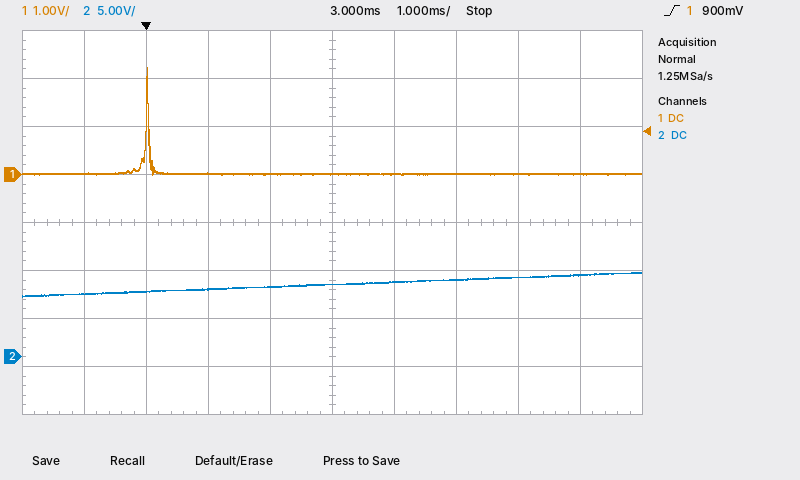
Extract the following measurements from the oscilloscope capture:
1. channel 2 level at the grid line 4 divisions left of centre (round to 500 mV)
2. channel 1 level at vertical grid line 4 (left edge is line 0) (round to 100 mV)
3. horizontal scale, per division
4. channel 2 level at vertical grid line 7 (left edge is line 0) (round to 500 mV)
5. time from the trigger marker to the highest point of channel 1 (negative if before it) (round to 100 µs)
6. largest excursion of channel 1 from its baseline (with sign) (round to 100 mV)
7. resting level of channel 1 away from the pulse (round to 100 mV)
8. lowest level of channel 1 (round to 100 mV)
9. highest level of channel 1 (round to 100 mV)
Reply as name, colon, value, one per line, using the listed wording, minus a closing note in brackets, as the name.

channel 2 level at the grid line 4 divisions left of centre: 6.5 V
channel 1 level at vertical grid line 4 (left edge is line 0): 0.0 V
horizontal scale, per division: 1 ms
channel 2 level at vertical grid line 7 (left edge is line 0): 8.0 V
time from the trigger marker to the highest point of channel 1 (negative if before it): 0.0 ms
largest excursion of channel 1 from its baseline (with sign): +2.2 V
resting level of channel 1 away from the pulse: 0.0 V
lowest level of channel 1: 0.0 V
highest level of channel 1: 2.2 V
